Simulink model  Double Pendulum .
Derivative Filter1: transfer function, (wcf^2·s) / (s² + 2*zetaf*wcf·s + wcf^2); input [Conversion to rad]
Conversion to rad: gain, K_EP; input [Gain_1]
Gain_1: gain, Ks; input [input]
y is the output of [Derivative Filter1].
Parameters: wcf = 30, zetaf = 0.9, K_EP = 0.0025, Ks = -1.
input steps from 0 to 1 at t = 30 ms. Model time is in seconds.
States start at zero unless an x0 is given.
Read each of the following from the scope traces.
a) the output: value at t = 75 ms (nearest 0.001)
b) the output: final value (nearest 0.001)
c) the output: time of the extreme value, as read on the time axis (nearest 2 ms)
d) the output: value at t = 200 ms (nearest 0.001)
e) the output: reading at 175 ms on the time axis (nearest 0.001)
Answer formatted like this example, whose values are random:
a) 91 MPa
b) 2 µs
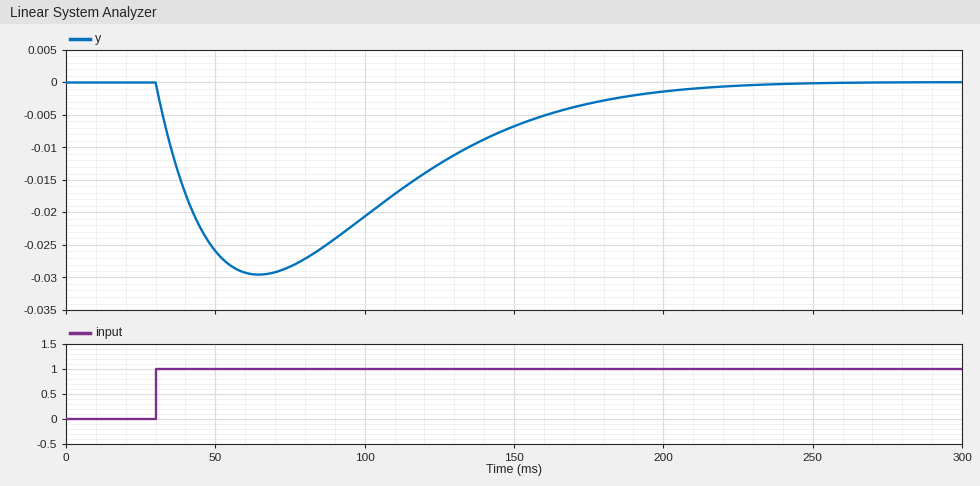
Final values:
a) -0.028
b) 0.000
c) 64 ms
d) -0.001
e) -0.003
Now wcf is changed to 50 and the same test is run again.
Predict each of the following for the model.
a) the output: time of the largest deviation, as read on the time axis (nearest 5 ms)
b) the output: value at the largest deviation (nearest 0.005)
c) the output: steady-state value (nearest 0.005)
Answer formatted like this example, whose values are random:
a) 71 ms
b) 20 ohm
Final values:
a) 50 ms
b) -0.050
c) 0.000
